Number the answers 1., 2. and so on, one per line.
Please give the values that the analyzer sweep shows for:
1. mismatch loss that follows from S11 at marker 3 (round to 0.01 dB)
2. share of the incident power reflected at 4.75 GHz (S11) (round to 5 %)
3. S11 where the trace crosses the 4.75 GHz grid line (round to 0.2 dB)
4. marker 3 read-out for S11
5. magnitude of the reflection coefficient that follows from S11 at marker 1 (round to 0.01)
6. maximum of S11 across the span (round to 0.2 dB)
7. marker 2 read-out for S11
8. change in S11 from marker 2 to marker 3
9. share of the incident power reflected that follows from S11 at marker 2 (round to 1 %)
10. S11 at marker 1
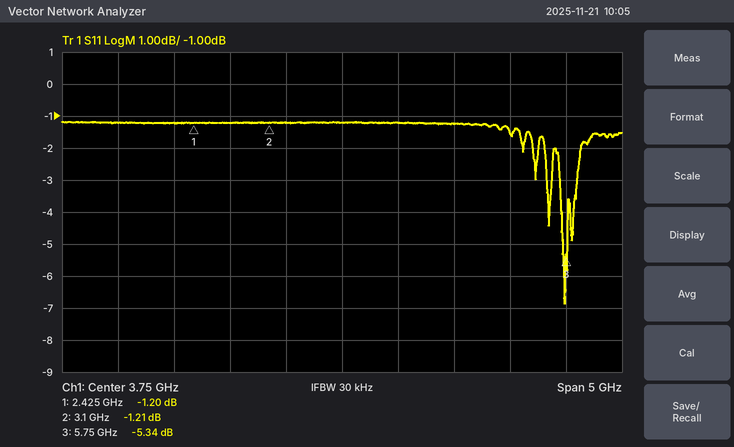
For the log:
1. 1.50 dB
2. 75 %
3. -1.2 dB
4. -5.34 dB
5. 0.87
6. -1.2 dB
7. -1.21 dB
8. -4.13 dB
9. 76 %
10. -1.20 dB
